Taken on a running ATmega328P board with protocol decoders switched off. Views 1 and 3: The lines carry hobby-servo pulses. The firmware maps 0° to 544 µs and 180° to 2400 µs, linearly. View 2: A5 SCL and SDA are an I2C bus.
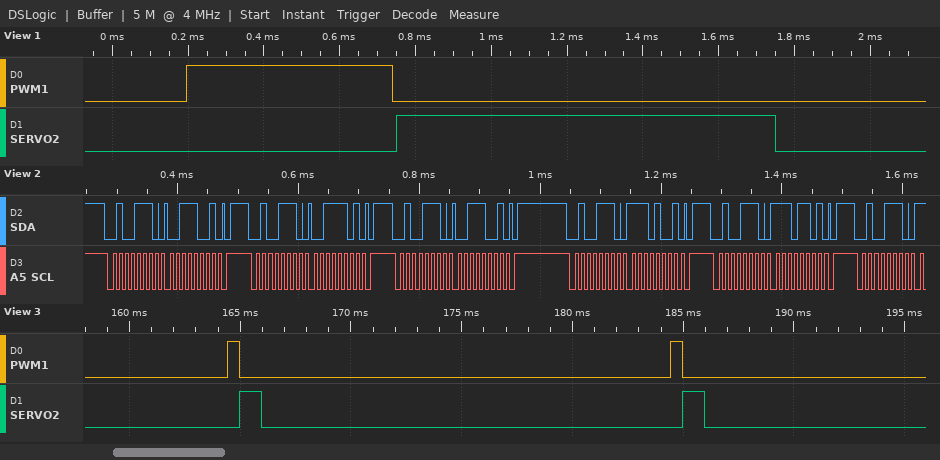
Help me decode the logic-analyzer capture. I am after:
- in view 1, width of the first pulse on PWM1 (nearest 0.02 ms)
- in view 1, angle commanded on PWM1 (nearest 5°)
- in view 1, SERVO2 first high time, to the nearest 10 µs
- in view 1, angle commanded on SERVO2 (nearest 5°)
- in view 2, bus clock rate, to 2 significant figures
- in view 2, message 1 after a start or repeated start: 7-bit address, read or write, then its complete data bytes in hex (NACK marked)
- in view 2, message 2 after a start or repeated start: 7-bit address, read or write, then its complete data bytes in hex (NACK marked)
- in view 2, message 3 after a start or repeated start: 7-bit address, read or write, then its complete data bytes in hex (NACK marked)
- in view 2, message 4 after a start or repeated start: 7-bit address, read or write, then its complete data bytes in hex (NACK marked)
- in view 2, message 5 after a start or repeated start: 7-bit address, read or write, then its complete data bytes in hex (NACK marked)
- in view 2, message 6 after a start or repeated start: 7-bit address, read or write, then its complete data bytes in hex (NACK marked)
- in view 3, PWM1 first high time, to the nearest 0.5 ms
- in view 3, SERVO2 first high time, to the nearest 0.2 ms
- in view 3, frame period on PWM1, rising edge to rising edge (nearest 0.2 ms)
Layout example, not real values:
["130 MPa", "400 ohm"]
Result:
["0.54 ms", "0°", "1000 µs", "45°", "100 kHz", "0x27 write: 39", "0x27 write: 3D", "0x27 write: 39", "0x27 write: E9", "0x27 write: ED", "0x27 write", "0.5 ms", "1.0 ms", "20.0 ms"]
